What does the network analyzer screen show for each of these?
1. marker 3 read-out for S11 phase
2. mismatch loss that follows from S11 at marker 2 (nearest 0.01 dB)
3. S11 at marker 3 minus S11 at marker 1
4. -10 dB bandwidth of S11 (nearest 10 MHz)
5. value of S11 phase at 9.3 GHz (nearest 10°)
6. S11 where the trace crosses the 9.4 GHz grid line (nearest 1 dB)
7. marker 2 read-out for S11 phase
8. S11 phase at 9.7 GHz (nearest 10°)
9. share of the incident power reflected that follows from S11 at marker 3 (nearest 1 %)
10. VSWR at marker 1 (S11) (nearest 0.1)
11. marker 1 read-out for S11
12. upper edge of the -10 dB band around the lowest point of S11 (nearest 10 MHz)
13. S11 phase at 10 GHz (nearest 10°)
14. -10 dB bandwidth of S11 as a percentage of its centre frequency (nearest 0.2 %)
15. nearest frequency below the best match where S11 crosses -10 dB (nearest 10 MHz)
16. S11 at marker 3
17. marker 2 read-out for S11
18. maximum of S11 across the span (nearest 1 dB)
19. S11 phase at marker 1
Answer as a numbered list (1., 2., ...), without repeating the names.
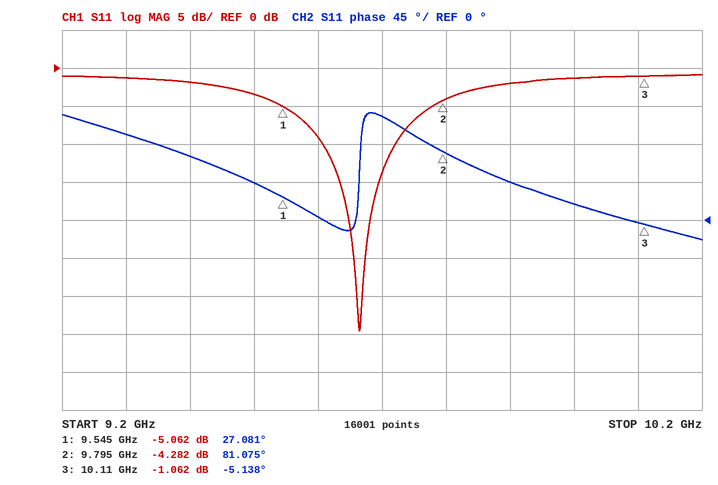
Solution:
1. -5.138°
2. 2.03 dB
3. 4.000 dB
4. 110 MHz
5. 100°
6. -2 dB
7. 81.075°
8. 120°
9. 78 %
10. 3.5
11. -5.062 dB
12. 9.72 GHz
13. 20°
14. 1.2 %
15. 9.61 GHz
16. -1.062 dB
17. -4.282 dB
18. -1 dB
19. 27.081°
